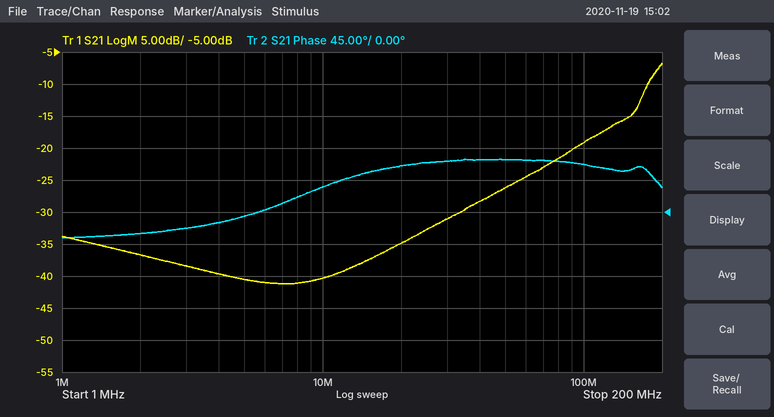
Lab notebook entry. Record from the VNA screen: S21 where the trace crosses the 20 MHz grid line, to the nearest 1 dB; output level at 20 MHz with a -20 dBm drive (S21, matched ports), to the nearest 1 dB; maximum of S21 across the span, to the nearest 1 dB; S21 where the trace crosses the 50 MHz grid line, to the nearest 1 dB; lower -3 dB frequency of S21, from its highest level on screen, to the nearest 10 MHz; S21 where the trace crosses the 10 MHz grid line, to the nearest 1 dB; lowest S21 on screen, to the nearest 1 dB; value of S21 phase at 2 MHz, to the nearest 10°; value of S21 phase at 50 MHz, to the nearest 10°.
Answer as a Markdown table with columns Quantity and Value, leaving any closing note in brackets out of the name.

| Quantity | Value |
|---|---|
| S21 where the trace crosses the 20 MHz grid line, to the nearest 1 dB | -35 dB |
| output level at 20 MHz with a -20 dBm drive (S21, matched ports), to the nearest 1 dB | -55 dBm |
| maximum of S21 across the span, to the nearest 1 dB | -7 dB |
| S21 where the trace crosses the 50 MHz grid line, to the nearest 1 dB | -26 dB |
| lower -3 dB frequency of S21, from its highest level on screen, to the nearest 10 MHz | 180 MHz |
| S21 where the trace crosses the 10 MHz grid line, to the nearest 1 dB | -40 dB |
| lowest S21 on screen, to the nearest 1 dB | -41 dB |
| value of S21 phase at 2 MHz, to the nearest 10° | -30° |
| value of S21 phase at 50 MHz, to the nearest 10° | 70° |
